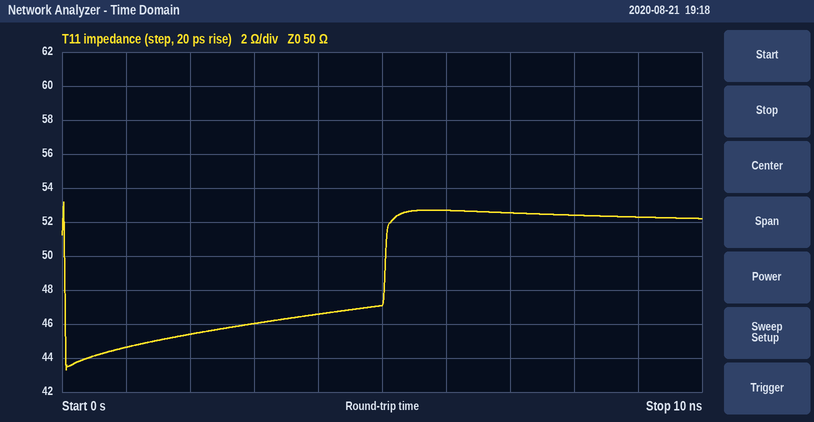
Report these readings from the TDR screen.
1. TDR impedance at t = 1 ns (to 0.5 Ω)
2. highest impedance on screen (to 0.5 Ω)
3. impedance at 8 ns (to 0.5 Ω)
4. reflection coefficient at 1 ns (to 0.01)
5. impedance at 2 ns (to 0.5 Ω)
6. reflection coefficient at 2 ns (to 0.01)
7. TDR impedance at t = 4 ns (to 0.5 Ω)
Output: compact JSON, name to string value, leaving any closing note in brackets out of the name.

{"TDR impedance at t = 1 ns": "44.5 Ω", "highest impedance on screen": "53.0 Ω", "impedance at 8 ns": "52.5 Ω", "reflection coefficient at 1 ns": "-0.06", "impedance at 2 ns": "45.5 Ω", "reflection coefficient at 2 ns": "-0.05", "TDR impedance at t = 4 ns": "46.5 Ω"}
